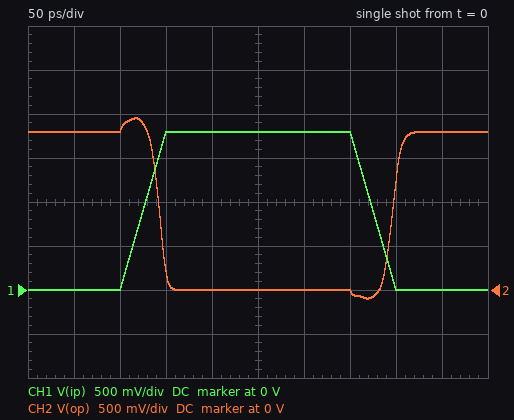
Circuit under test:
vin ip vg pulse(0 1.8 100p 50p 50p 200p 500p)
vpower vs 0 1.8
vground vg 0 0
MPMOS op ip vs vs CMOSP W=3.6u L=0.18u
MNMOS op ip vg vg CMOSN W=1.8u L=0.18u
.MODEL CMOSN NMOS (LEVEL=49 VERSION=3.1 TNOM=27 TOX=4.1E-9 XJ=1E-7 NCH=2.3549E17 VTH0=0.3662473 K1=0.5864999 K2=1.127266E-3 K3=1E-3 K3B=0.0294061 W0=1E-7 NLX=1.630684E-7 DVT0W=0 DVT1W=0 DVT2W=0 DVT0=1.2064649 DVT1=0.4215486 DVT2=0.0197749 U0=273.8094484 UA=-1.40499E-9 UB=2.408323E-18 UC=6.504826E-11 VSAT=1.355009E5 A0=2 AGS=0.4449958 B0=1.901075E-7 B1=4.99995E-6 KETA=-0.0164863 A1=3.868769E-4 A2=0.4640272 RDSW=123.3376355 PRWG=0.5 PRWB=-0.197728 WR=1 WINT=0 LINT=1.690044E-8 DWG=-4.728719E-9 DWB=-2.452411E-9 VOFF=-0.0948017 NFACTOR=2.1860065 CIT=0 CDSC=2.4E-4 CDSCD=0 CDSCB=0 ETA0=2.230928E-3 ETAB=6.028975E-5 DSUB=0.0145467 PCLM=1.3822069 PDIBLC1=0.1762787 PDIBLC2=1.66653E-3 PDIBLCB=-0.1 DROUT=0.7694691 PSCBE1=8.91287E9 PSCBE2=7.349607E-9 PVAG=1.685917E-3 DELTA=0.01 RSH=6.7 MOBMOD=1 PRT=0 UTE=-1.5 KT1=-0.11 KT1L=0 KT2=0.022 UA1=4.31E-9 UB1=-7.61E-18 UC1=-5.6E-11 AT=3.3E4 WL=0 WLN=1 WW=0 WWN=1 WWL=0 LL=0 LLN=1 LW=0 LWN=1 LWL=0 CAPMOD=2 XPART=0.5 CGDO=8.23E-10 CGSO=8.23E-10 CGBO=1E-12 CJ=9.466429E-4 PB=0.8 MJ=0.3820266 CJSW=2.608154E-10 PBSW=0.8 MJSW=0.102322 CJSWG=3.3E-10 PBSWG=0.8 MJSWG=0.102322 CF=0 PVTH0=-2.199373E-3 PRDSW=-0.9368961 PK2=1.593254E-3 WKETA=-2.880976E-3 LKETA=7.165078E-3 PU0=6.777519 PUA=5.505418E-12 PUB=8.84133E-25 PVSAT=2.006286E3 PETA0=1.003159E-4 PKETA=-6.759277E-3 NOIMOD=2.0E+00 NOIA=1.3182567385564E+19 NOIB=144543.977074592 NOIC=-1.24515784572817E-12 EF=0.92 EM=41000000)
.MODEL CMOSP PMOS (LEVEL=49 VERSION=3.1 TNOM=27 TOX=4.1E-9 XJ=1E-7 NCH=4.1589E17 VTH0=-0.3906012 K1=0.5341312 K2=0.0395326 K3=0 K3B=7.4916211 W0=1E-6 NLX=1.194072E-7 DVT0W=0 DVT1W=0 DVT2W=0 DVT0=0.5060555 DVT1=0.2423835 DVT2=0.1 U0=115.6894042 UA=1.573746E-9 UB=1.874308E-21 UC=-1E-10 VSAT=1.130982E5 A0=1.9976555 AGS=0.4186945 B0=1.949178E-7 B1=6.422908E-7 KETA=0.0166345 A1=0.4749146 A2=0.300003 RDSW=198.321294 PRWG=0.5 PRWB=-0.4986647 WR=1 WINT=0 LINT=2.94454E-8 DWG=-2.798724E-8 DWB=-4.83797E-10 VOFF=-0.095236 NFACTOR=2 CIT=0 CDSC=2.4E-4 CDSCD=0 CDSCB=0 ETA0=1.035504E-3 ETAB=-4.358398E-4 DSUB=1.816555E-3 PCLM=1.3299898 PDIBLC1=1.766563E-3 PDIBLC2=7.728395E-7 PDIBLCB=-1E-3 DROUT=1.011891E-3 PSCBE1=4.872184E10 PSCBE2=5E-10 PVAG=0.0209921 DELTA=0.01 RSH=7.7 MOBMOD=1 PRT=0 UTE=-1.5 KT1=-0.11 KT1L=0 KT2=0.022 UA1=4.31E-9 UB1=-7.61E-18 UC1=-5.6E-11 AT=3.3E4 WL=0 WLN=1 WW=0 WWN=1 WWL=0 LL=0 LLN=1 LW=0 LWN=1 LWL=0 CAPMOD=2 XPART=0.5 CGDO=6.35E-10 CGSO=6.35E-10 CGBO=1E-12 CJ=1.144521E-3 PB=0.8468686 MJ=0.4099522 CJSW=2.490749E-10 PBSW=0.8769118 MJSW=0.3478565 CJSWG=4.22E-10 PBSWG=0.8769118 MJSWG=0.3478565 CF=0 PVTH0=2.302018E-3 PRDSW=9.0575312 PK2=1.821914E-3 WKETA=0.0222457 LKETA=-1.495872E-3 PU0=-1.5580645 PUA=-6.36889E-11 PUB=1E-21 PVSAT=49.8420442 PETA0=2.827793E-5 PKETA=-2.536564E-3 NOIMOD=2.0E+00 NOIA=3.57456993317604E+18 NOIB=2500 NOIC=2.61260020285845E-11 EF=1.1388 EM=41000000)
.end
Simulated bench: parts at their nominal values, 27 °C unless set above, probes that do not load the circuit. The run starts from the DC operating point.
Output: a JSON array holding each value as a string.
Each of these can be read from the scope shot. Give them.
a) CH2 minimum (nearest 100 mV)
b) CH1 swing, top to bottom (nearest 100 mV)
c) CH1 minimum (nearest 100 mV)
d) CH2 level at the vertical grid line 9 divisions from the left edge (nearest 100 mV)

["-100 mV", "1.8 V", "0 V", "1.8 V"]
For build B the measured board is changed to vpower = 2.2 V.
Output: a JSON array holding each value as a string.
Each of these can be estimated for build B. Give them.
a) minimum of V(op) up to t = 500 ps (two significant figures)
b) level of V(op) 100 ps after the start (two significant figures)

["-76 mV", "2.2 V"]
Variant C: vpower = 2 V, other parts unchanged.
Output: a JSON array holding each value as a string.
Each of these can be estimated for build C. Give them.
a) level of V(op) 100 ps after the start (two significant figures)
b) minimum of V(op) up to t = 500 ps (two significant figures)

["2.0 V", "-85 mV"]
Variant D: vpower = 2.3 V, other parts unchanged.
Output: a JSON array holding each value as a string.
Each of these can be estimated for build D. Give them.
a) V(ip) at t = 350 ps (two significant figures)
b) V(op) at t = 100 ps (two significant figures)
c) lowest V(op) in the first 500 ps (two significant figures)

["1.8 V", "2.3 V", "-69 mV"]
